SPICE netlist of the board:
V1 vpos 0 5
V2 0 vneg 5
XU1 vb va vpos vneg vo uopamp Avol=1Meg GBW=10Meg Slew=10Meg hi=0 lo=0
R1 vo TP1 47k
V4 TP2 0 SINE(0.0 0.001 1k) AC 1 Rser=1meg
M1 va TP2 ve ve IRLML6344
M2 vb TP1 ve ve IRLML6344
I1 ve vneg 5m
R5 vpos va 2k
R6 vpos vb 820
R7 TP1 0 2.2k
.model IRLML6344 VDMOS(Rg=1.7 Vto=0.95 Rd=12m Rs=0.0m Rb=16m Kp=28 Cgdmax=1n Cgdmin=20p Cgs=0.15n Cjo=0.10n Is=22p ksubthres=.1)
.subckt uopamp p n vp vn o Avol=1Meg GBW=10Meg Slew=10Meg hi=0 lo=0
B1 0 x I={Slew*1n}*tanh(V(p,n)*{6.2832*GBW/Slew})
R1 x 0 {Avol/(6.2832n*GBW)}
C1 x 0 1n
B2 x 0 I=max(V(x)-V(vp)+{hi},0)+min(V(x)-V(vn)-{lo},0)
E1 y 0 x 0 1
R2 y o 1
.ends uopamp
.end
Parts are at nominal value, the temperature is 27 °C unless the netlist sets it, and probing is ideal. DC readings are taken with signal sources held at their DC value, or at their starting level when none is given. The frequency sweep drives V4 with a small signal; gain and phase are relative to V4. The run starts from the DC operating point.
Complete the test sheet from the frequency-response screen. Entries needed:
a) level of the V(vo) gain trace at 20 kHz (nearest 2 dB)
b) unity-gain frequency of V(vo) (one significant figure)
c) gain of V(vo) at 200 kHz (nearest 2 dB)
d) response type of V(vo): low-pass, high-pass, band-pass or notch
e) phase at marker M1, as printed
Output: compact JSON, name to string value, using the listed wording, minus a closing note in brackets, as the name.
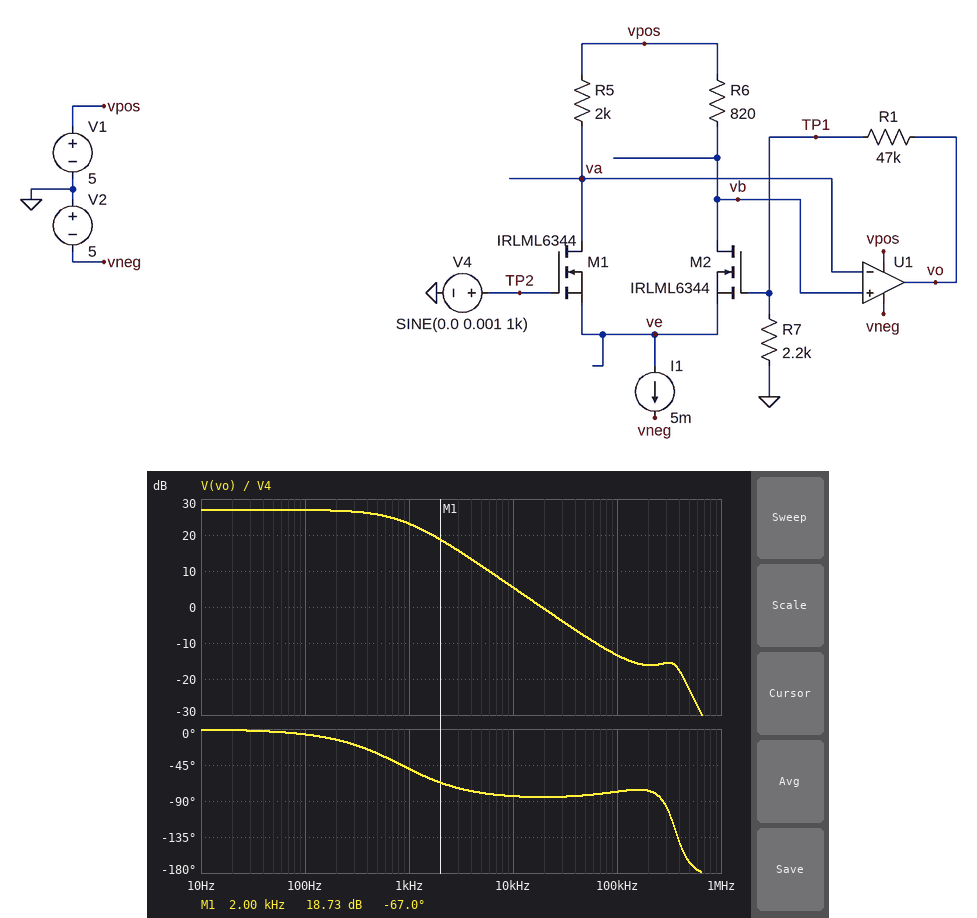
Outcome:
{"level of the V(vo) gain trace at 20 kHz": "0 dB", "unity-gain frequency of V(vo)": "20 kHz", "gain of V(vo) at 200 kHz": "-16 dB", "response type of V(vo): low-pass, high-pass, band-pass or notch": "low-pass", "phase at marker M1, as printed": "-67.0 deg"}
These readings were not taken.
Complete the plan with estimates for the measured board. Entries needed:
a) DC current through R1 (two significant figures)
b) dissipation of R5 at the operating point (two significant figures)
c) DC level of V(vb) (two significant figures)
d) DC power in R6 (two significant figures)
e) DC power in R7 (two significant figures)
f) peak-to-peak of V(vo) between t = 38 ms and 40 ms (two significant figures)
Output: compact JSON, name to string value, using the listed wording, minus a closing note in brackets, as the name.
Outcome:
{"DC current through R1": "22 µA", "dissipation of R5 at the operating point": "4.2 mW", "DC level of V(vb)": "2.1 V", "DC power in R6": "10 mW", "DC power in R7": "1.0 µW", "peak-to-peak of V(vo) between t = 38 ms and 40 ms": "29 mV"}
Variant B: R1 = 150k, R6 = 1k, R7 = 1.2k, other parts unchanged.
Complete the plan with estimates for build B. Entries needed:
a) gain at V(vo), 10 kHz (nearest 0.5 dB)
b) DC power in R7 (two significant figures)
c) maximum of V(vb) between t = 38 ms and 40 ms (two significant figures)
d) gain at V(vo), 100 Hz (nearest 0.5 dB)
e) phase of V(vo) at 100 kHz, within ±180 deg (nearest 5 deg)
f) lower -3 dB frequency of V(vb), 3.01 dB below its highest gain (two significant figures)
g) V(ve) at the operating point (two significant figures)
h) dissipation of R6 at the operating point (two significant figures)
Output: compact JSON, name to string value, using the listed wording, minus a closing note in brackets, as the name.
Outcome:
{"gain at V(vo), 10 kHz": "19.0 dB", "DC power in R7": "1.1 µW", "maximum of V(vb) between t = 38 ms and 40 ms": "1.7 V", "gain at V(vo), 100 Hz": "42.0 dB", "phase of V(vo) at 100 kHz, within ±180 deg": "-125 deg", "lower -3 dB frequency of V(vb), 3.01 dB below its highest gain": "710 Hz", "V(ve) at the operating point": "-730 mV", "dissipation of R6 at the operating point": "11 mW"}
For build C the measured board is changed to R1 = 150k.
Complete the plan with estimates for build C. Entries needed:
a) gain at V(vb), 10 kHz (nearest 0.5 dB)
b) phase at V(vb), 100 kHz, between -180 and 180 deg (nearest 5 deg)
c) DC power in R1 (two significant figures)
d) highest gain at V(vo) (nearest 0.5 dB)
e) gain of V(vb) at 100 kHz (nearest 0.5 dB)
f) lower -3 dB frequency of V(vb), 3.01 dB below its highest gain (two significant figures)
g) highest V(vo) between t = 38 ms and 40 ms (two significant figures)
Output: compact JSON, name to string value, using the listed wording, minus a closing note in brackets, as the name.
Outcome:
{"gain at V(vb), 10 kHz": "-51.0 dB", "phase at V(vb), 100 kHz, between -180 and 180 deg": "-15 deg", "DC power in R1": "70 µW", "highest gain at V(vo)": "37.0 dB", "gain of V(vb) at 100 kHz": "-50.0 dB", "lower -3 dB frequency of V(vb), 3.01 dB below its highest gain": "1.2 kHz", "highest V(vo) between t = 38 ms and 40 ms": "3.3 V"}
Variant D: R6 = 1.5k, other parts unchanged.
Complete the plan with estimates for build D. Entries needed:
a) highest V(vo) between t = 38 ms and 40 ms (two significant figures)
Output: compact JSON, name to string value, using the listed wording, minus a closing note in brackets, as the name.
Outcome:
{"highest V(vo) between t = 38 ms and 40 ms": "350 mV"}
